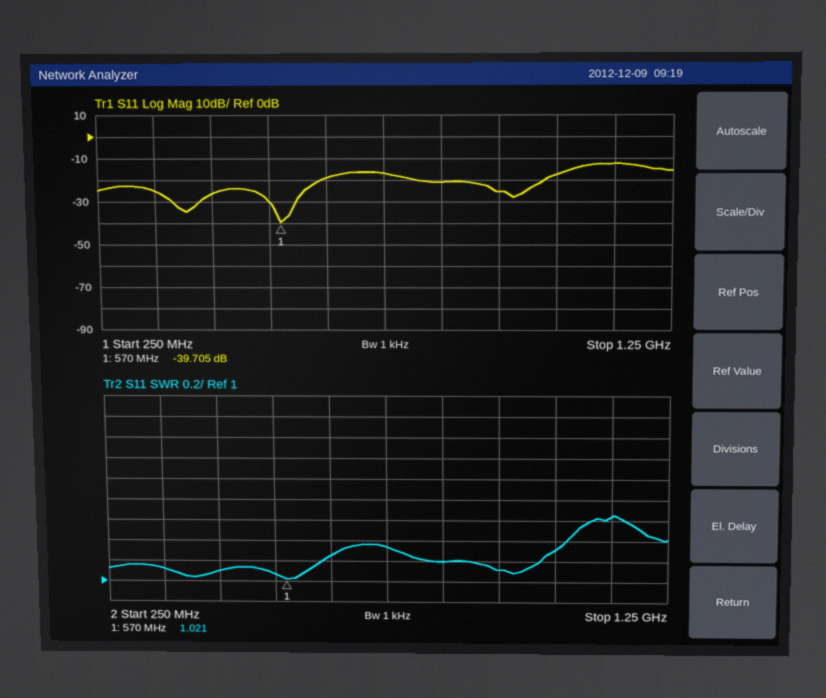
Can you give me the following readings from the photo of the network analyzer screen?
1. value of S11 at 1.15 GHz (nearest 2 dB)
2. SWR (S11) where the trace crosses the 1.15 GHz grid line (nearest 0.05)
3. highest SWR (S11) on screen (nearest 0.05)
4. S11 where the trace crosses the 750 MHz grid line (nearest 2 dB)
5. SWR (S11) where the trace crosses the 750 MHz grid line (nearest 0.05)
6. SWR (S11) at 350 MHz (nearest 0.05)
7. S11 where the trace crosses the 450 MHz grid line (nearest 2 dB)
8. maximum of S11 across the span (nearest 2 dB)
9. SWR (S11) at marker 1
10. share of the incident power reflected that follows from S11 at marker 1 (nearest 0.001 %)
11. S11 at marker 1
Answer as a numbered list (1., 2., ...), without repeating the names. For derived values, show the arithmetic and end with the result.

1. -12 dB
2. 1.65
3. 1.65
4. -16 dB
5. 1.35
6. 1.10
7. -26 dB
8. -12 dB
9. 1.021
10. 10^(-39.705/10) ≈ 0.011 %
11. -39.705 dB
